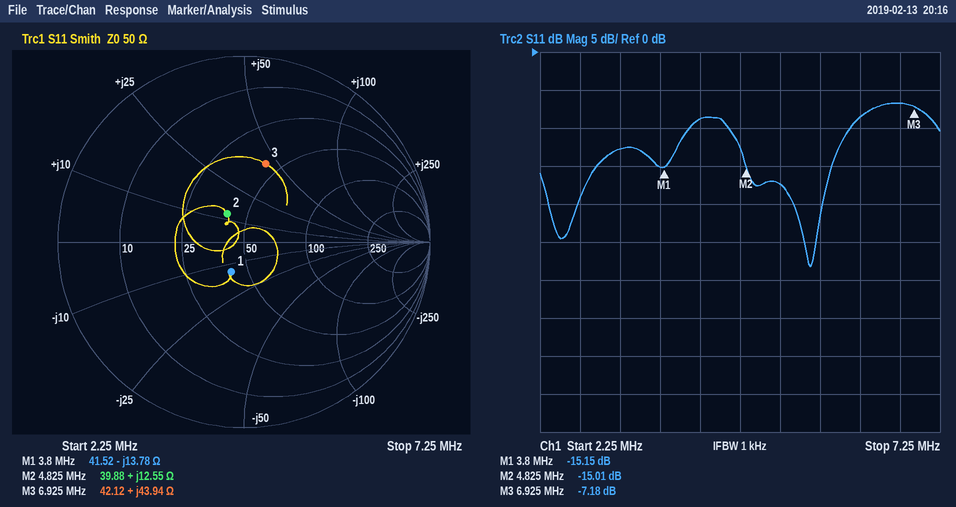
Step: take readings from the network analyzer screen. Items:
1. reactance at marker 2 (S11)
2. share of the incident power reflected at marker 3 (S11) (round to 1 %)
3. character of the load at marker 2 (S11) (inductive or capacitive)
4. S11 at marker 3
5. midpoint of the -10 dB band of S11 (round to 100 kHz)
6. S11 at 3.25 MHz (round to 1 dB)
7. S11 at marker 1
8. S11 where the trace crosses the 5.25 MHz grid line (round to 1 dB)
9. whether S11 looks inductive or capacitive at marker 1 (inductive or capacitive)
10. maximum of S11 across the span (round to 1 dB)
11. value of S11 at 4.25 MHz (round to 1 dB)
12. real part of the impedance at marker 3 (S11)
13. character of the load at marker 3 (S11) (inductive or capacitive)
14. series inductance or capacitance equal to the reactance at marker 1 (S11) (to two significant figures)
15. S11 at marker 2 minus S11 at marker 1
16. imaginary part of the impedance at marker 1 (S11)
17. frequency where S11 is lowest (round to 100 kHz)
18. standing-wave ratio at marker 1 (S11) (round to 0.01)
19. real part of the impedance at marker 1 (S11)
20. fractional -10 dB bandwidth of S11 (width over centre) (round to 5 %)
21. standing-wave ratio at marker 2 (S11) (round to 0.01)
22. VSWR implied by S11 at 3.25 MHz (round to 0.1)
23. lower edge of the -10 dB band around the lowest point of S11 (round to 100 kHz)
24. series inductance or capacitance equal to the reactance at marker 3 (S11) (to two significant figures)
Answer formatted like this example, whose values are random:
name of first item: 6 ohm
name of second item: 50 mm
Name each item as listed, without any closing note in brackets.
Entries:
reactance at marker 2: +12.55 Ω
share of the incident power reflected at marker 3 (S11): 19 %
character of the load at marker 2 (S11): inductive
S11 at marker 3: -7.18 dB
midpoint of the -10 dB band of S11: 5.4 MHz
S11 at 3.25 MHz: -13 dB
S11 at marker 1: -15.15 dB
S11 where the trace crosses the 5.25 MHz grid line: -17 dB
whether S11 looks inductive or capacitive at marker 1: capacitive
maximum of S11 across the span: -7 dB
value of S11 at 4.25 MHz: -9 dB
real part of the impedance at marker 3: 42.12 Ω
character of the load at marker 3 (S11): inductive
series inductance or capacitance equal to the reactance at marker 1 (S11): 3.0 nF
S11 at marker 2 minus S11 at marker 1: 0.14 dB
imaginary part of the impedance at marker 1: -13.78 Ω
frequency where S11 is lowest: 5.6 MHz
standing-wave ratio at marker 1 (S11): 1.42
real part of the impedance at marker 1: 41.52 Ω
fractional -10 dB bandwidth of S11 (width over centre): 30 %
standing-wave ratio at marker 2 (S11): 1.43
VSWR implied by S11 at 3.25 MHz: 1.6
lower edge of the -10 dB band around the lowest point of S11: 4.6 MHz
series inductance or capacitance equal to the reactance at marker 3 (S11): 1.0 µH
